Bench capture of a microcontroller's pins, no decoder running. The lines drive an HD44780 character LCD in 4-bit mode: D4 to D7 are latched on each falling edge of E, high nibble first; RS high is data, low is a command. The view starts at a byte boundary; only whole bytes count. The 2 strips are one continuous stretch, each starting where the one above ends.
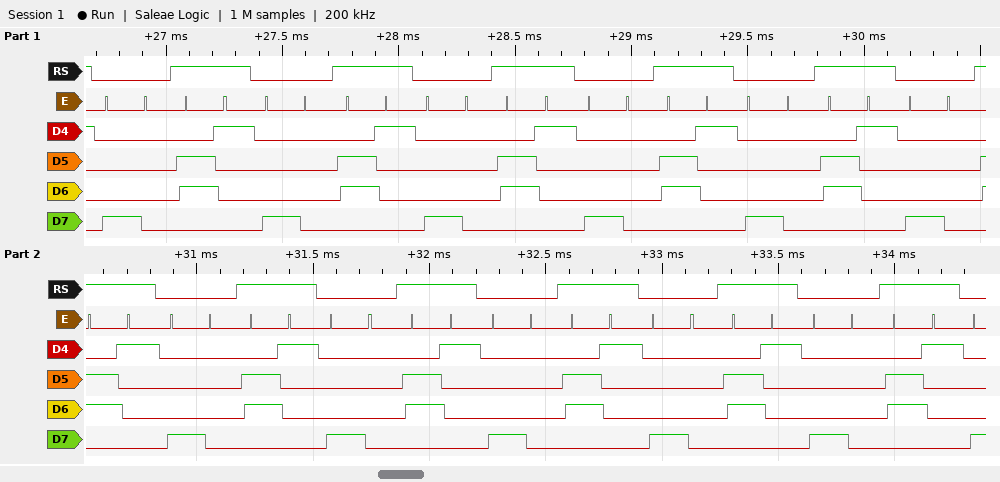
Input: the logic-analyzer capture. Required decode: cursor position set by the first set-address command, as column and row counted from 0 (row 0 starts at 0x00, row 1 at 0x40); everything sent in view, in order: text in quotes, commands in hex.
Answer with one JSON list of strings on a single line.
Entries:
["column 0, row 0", "0x80 \"a\" 0x80 \"a\" 0x80 \"a\" 0x80 \"a\" 0x80 \"a\" 0x80 \"a\" 0x80 \"a\" 0x80 \"a\" 0x80 \"a\" 0x80 \"a\" 0x80 \"a\""]
